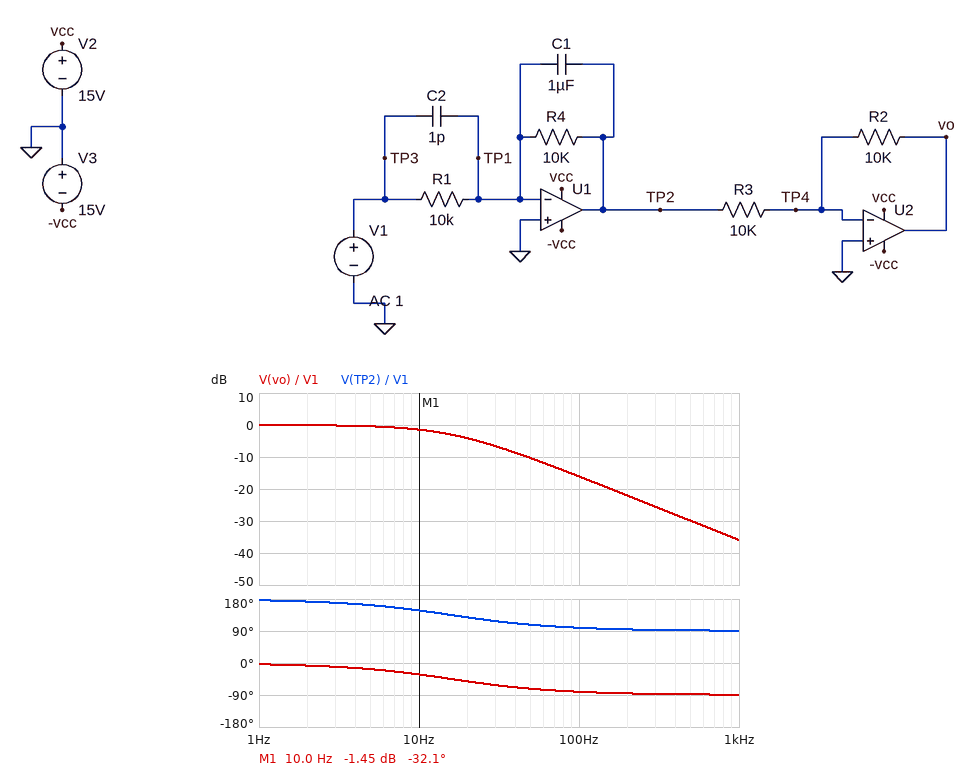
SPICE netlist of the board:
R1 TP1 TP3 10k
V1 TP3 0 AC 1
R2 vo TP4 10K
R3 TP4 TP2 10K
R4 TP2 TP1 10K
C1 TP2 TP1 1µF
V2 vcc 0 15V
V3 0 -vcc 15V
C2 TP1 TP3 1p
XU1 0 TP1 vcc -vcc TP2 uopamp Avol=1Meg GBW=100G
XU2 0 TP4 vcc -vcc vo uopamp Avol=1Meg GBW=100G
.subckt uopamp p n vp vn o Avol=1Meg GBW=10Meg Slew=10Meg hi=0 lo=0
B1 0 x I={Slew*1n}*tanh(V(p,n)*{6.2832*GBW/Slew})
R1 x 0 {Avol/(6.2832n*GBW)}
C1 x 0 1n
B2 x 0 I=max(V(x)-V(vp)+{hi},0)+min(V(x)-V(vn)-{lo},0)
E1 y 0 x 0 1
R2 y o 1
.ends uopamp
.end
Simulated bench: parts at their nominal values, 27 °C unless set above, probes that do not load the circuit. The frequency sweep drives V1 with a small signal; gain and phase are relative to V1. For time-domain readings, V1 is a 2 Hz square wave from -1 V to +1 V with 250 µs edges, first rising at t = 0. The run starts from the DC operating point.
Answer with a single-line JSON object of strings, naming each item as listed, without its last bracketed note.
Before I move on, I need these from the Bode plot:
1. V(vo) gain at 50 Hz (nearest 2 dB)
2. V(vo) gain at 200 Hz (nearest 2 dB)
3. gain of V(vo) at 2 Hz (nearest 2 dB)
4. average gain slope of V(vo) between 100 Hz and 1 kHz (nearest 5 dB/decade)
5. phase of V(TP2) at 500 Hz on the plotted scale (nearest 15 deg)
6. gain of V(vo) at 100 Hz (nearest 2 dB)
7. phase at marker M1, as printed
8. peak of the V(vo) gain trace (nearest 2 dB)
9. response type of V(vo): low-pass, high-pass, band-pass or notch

{"V(vo) gain at 50 Hz": "-10 dB", "V(vo) gain at 200 Hz": "-22 dB", "gain of V(vo) at 2 Hz": "0 dB", "average gain slope of V(vo) between 100 Hz and 1 kHz": "-20 dB/decade", "phase of V(TP2) at 500 Hz on the plotted scale": "90 deg", "gain of V(vo) at 100 Hz": "-16 dB", "phase at marker M1, as printed": "-32.1 deg", "peak of the V(vo) gain trace": "0 dB", "response type of V(vo): low-pass, high-pass, band-pass or notch": "low-pass"}
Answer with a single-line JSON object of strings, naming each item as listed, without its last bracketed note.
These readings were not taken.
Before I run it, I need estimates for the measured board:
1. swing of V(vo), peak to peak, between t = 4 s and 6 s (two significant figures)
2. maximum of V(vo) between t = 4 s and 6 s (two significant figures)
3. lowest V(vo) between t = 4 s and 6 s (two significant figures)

{"swing of V(vo), peak to peak, between t = 4 s and 6 s": "2.0 V", "maximum of V(vo) between t = 4 s and 6 s": "1.0 V", "lowest V(vo) between t = 4 s and 6 s": "-1.0 V"}
